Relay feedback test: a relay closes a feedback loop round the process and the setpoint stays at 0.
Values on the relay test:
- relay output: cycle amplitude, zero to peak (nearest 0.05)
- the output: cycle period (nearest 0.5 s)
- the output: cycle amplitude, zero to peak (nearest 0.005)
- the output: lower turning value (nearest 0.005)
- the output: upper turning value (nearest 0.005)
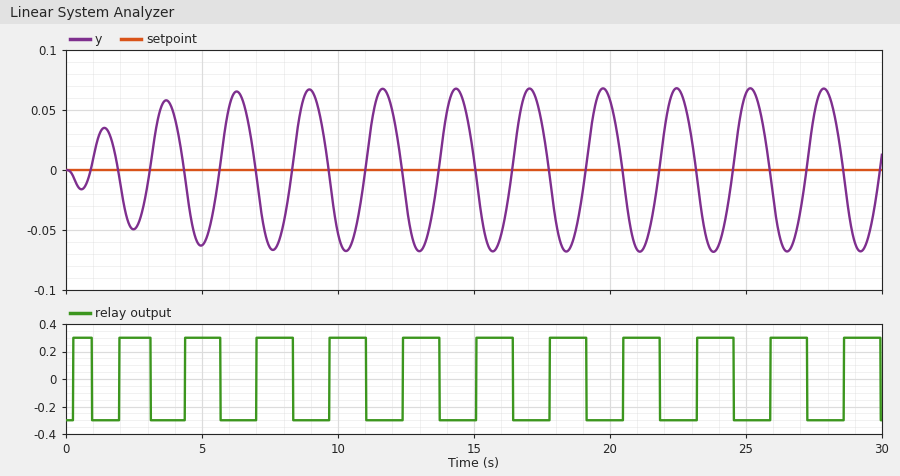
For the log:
0.30
2.5 s
0.070
-0.070
0.070
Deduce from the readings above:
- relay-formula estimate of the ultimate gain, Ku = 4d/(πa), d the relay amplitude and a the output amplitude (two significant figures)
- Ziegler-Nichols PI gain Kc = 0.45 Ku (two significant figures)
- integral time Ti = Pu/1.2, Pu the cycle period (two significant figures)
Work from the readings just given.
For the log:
5.5
2.5
2.1 s
